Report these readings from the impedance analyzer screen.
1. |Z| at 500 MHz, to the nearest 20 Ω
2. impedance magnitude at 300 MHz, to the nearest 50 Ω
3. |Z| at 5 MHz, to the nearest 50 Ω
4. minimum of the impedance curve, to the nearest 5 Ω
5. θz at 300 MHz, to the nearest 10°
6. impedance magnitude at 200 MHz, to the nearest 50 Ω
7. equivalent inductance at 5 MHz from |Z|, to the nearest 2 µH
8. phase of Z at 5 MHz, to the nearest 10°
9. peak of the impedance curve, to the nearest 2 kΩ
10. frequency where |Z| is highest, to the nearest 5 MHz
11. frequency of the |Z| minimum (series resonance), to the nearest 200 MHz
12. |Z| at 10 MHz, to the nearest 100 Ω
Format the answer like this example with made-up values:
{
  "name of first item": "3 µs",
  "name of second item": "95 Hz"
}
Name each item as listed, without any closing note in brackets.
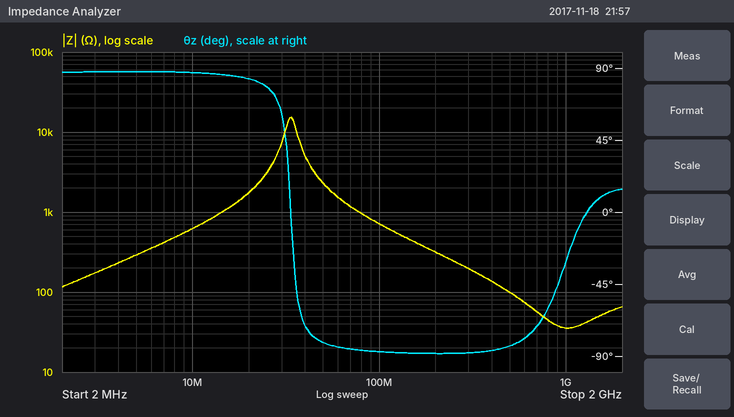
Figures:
{
  "|Z| at 500 MHz, to the nearest 20 Ω": "100 Ω",
  "impedance magnitude at 300 MHz, to the nearest 50 Ω": "200 Ω",
  "|Z| at 5 MHz, to the nearest 50 Ω": "300 Ω",
  "minimum of the impedance curve, to the nearest 5 Ω": "35 Ω",
  "θz at 300 MHz, to the nearest 10°": "-90°",
  "impedance magnitude at 200 MHz, to the nearest 50 Ω": "300 Ω",
  "equivalent inductance at 5 MHz from |Z|, to the nearest 2 µH": "10 µH",
  "phase of Z at 5 MHz, to the nearest 10°": "90°",
  "peak of the impedance curve, to the nearest 2 kΩ": "16 kΩ",
  "frequency where |Z| is highest, to the nearest 5 MHz": "35 MHz",
  "frequency of the |Z| minimum (series resonance), to the nearest 200 MHz": "1.0 GHz",
  "|Z| at 10 MHz, to the nearest 100 Ω": "600 Ω"
}
